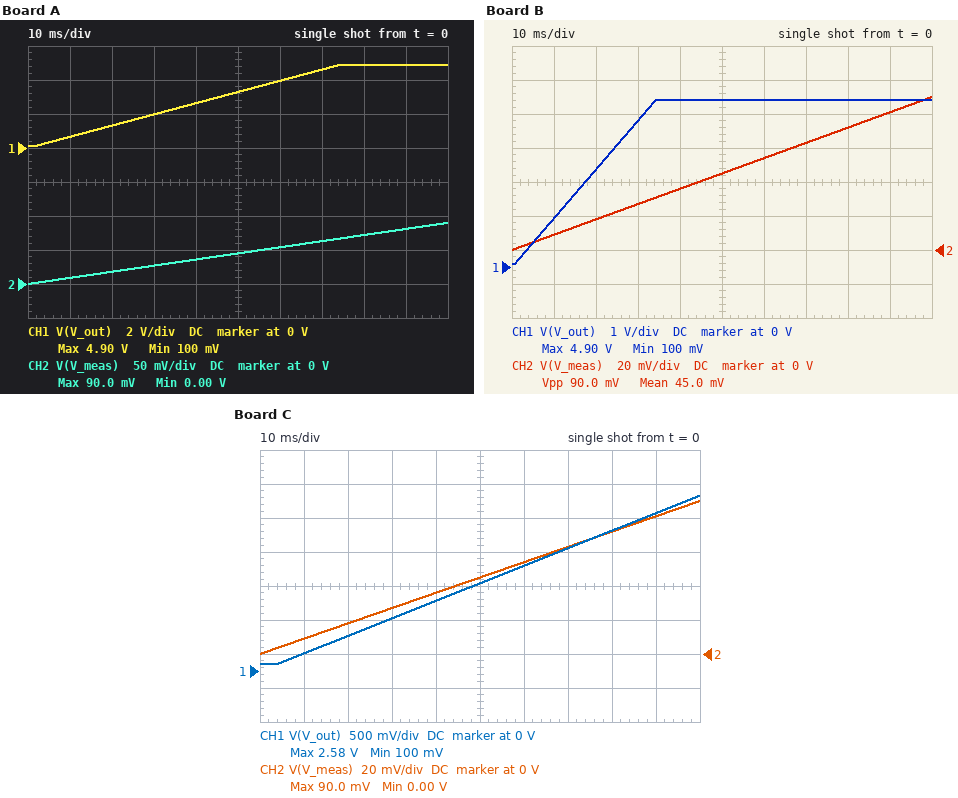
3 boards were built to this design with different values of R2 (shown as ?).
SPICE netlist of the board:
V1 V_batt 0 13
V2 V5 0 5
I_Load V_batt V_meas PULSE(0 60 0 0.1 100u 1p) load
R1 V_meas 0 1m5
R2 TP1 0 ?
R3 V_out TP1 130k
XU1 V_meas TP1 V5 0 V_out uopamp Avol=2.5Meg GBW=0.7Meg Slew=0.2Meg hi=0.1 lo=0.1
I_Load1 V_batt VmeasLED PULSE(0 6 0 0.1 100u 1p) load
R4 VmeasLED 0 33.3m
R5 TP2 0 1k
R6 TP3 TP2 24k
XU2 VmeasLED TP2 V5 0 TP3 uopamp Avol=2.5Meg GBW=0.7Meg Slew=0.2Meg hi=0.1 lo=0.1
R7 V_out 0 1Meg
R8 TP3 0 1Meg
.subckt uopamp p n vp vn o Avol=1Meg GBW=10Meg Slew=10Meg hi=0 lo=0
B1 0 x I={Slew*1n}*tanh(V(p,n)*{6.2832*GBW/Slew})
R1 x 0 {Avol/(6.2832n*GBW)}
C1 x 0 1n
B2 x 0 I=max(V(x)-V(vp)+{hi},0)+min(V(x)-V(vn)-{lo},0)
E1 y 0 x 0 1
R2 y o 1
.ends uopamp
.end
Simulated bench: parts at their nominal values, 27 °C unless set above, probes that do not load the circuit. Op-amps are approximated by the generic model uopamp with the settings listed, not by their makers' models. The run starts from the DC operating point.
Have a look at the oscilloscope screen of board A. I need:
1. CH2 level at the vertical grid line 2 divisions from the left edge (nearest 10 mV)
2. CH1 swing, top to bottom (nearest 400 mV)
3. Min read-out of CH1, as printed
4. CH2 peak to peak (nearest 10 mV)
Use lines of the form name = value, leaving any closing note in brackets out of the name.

CH2 level at the vertical grid line 2 divisions from the left edge = 20 mV
CH1 swing, top to bottom = 4.8 V
Min read-out of CH1, as printed = 100 mV
CH2 peak to peak = 90 mV
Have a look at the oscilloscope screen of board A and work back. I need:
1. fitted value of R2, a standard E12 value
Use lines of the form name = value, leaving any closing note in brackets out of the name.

fitted value of R2, a standard E12 value = 1.8 kΩ
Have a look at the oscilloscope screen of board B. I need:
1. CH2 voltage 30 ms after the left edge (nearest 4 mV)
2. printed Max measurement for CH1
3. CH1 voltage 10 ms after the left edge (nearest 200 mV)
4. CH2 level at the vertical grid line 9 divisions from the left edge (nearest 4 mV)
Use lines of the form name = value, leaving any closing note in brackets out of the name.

CH2 voltage 30 ms after the left edge = 28 mV
printed Max measurement for CH1 = 4.90 V
CH1 voltage 10 ms after the left edge = 1.4 V
CH2 level at the vertical grid line 9 divisions from the left edge = 80 mV
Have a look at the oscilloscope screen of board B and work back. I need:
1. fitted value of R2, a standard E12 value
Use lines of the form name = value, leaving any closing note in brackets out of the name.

fitted value of R2, a standard E12 value = 820 Ω
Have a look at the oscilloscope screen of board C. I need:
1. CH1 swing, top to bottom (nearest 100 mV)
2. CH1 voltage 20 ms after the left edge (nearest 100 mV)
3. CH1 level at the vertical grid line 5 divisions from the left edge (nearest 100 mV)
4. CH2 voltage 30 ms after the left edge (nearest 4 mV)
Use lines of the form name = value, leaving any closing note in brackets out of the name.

CH1 swing, top to bottom = 2.5 V
CH1 voltage 20 ms after the left edge = 500 mV
CH1 level at the vertical grid line 5 divisions from the left edge = 1.3 V
CH2 voltage 30 ms after the left edge = 28 mV
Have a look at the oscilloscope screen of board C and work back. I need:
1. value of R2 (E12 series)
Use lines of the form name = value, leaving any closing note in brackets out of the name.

value of R2 = 4.7 kΩ
